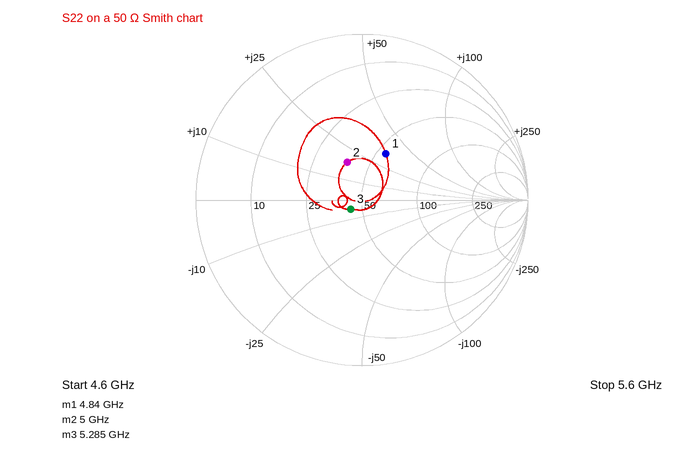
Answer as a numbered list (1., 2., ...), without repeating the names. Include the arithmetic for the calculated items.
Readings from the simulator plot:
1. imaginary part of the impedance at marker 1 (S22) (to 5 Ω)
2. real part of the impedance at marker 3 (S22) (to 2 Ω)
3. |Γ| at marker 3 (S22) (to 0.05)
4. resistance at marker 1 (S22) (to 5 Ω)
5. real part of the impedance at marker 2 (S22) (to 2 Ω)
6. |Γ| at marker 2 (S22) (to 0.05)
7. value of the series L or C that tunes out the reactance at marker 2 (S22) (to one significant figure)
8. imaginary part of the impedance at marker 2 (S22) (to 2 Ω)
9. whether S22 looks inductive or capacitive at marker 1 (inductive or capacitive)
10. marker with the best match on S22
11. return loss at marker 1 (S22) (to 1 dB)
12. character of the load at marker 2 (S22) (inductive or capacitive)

1. +35 Ω
2. 44 Ω
3. 0.10
4. 55 Ω
5. 38 Ω
6. 0.25
7. C = 1/(2π × 5 GHz × 18 Ω) ≈ 2 pF
8. +18 Ω
9. inductive
10. marker 3
11. 10 dB
12. inductive
